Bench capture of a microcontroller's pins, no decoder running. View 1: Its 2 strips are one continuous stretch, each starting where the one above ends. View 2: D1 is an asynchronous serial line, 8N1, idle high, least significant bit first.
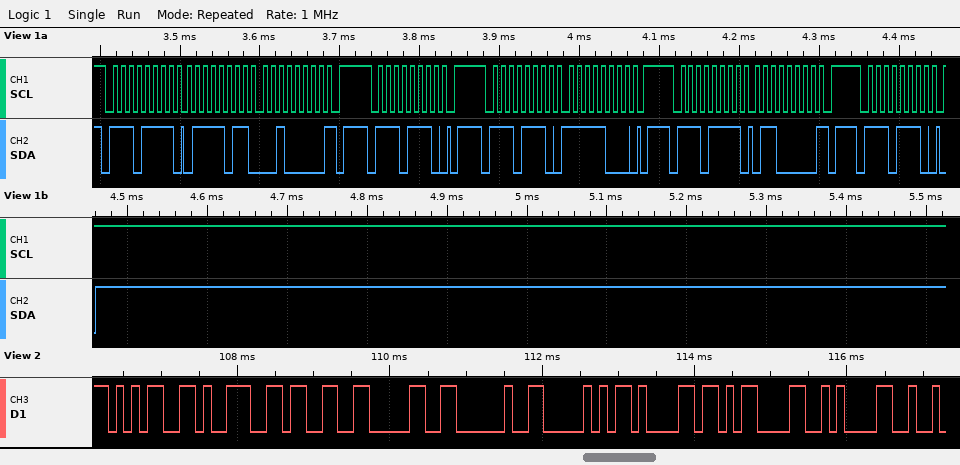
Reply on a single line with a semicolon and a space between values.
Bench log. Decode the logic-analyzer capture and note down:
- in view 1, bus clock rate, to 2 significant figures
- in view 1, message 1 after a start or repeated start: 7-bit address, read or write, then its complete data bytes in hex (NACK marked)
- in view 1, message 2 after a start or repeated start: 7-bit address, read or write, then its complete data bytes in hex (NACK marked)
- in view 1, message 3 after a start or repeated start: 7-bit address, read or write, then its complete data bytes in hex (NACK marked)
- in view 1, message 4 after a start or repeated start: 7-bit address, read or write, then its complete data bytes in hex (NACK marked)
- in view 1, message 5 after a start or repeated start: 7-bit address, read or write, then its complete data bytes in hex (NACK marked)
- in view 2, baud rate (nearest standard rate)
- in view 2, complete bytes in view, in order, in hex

100 kHz; 0x77 read: 7B 20 NACK; 0x77 write; 0x77 write: F8; 0x77 read: 60 NACK; 0x77 write; 9600 baud; 35 39 33 30 20 50 61 0D 0A
